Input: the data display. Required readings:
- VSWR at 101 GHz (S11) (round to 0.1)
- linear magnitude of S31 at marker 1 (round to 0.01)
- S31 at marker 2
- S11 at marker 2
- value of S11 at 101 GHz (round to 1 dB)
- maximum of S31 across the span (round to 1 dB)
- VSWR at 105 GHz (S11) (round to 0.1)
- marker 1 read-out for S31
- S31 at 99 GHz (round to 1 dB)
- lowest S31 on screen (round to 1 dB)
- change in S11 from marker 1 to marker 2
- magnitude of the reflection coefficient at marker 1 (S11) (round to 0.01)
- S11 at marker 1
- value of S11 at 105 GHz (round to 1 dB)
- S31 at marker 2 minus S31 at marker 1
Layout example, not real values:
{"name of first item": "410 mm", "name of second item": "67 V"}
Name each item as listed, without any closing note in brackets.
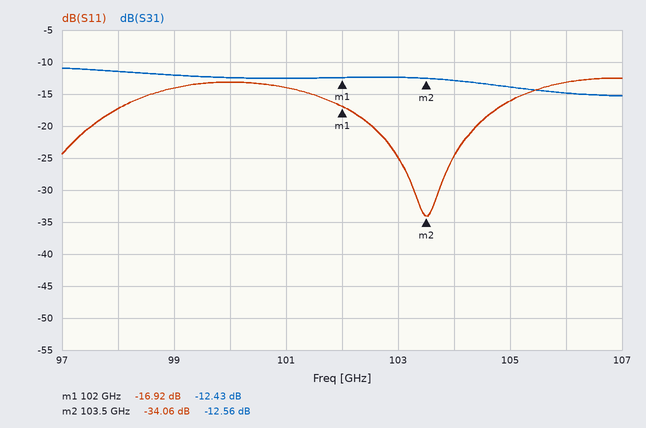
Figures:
{"VSWR at 101 GHz (S11)": "1.5", "linear magnitude of S31 at marker 1": "0.24", "S31 at marker 2": "-12.56 dB", "S11 at marker 2": "-34.06 dB", "value of S11 at 101 GHz": "-14 dB", "maximum of S31 across the span": "-11 dB", "VSWR at 105 GHz (S11)": "1.4", "marker 1 read-out for S31": "-12.43 dB", "S31 at 99 GHz": "-12 dB", "lowest S31 on screen": "-15 dB", "change in S11 from marker 1 to marker 2": "-17.14 dB", "magnitude of the reflection coefficient at marker 1 (S11)": "0.14", "S11 at marker 1": "-16.92 dB", "value of S11 at 105 GHz": "-16 dB", "S31 at marker 2 minus S31 at marker 1": "-0.13 dB"}
